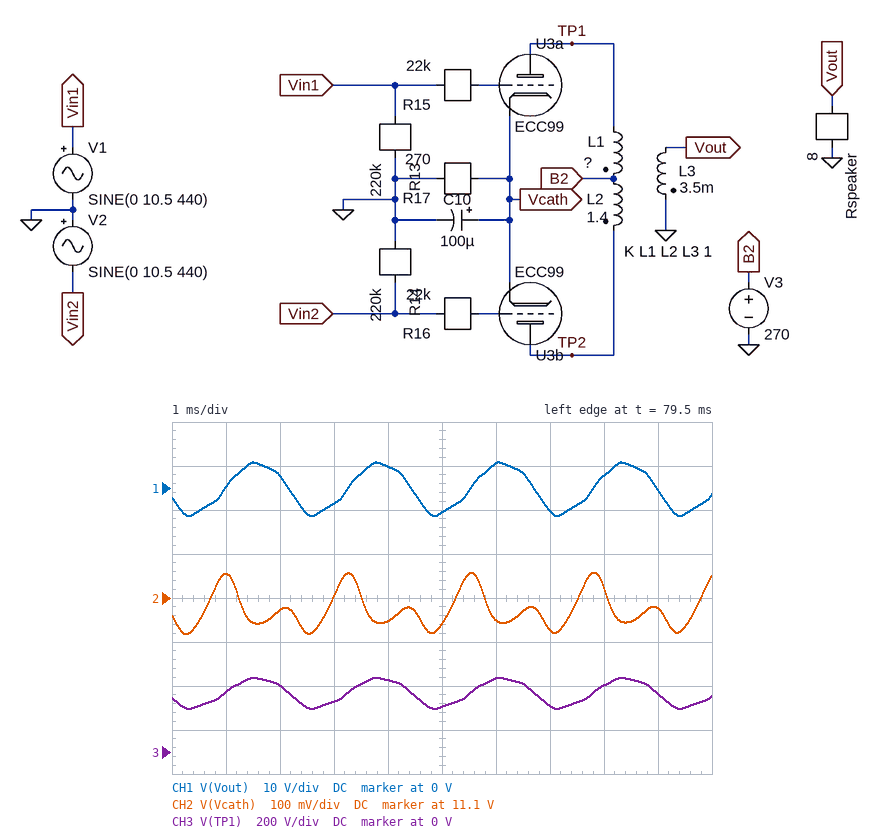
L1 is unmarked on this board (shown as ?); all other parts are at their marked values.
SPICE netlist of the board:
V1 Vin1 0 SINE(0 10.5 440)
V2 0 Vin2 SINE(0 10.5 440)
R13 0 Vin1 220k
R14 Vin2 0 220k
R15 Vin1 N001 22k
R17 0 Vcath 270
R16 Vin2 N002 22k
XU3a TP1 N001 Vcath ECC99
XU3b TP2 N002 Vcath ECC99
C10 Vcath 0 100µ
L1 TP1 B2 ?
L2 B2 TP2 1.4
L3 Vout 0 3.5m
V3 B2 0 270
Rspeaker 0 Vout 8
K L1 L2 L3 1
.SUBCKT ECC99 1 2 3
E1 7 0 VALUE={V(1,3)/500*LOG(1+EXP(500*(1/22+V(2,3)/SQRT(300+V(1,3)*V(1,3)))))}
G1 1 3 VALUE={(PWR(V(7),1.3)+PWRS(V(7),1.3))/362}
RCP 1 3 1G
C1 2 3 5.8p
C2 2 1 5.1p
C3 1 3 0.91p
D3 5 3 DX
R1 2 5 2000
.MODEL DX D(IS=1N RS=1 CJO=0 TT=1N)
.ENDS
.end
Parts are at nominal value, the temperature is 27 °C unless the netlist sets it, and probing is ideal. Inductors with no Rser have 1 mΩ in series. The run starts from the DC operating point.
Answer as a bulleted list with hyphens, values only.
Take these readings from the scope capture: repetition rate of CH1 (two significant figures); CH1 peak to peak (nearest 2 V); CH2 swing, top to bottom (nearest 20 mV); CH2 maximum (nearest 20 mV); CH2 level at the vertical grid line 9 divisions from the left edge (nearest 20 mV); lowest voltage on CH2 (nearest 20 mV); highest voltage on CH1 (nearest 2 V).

- 440 Hz
- 12 V
- 140 mV
- 11.16 V
- 11.08 V
- 11.02 V
- 6 V
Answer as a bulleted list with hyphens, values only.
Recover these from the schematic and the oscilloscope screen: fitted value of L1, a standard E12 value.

- 470 mH
